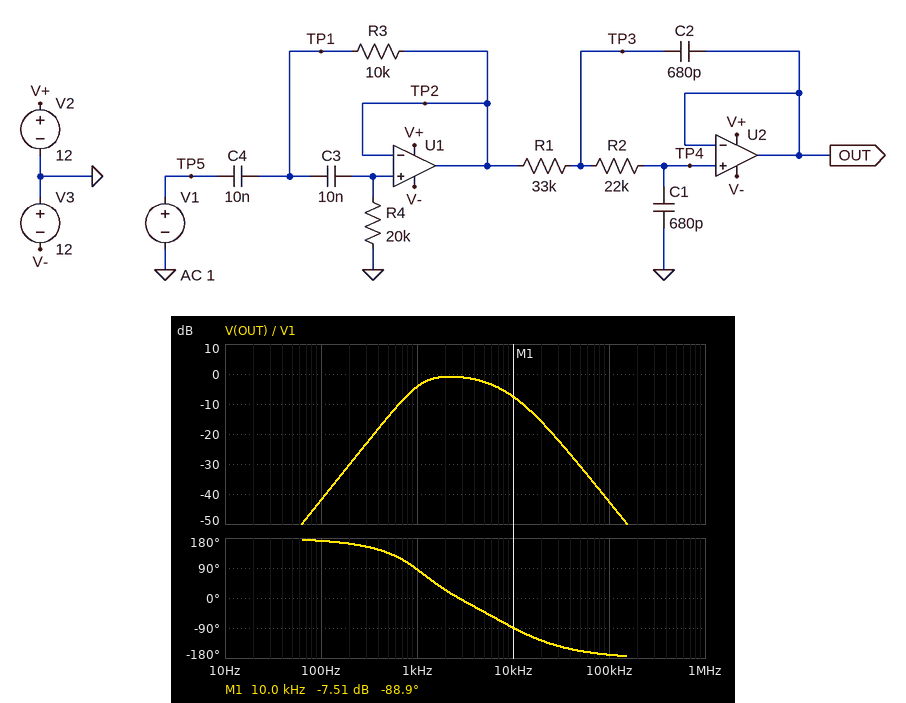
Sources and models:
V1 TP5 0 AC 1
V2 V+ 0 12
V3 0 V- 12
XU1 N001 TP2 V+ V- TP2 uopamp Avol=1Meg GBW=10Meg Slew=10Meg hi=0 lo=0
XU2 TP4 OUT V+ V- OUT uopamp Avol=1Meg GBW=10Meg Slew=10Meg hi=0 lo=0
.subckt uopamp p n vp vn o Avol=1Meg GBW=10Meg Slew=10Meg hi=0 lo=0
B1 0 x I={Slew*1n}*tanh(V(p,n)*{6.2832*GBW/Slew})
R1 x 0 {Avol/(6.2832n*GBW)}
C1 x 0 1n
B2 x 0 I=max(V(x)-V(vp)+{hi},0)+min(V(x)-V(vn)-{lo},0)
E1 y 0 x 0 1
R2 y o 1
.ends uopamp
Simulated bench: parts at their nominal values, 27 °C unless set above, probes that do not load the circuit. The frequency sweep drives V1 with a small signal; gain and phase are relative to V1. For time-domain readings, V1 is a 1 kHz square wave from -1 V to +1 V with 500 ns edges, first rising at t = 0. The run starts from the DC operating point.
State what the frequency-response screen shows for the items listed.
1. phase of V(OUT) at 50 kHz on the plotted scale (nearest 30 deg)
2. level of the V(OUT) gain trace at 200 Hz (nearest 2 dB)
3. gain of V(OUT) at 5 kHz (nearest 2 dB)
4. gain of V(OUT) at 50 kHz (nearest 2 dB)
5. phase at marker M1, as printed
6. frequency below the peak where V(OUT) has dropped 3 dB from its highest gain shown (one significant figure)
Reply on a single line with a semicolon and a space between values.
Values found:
-150 deg; -30 dB; -2 dB; -30 dB; -88.9 deg; 1 kHz
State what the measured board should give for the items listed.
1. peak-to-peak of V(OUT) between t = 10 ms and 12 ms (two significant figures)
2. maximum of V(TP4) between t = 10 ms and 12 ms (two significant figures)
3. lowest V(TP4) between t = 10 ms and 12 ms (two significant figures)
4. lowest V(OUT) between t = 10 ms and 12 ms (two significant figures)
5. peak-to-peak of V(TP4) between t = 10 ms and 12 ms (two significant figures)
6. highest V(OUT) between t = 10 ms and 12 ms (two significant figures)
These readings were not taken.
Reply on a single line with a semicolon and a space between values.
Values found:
2.8 V; 1.4 V; -1.4 V; -1.4 V; 2.8 V; 1.4 V
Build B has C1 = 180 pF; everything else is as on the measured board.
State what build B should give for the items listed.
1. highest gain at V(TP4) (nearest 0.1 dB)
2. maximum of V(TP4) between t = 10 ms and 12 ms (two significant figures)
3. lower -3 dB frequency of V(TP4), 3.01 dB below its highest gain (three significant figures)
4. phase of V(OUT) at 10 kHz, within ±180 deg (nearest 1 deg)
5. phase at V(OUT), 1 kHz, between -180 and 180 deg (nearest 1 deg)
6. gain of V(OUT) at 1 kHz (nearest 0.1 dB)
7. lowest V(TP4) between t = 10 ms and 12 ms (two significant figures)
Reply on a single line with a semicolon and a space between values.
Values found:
1.0 dB; 2.1 V; 1.28 kHz; -35 deg; 96 deg; -4.1 dB; -2.1 V
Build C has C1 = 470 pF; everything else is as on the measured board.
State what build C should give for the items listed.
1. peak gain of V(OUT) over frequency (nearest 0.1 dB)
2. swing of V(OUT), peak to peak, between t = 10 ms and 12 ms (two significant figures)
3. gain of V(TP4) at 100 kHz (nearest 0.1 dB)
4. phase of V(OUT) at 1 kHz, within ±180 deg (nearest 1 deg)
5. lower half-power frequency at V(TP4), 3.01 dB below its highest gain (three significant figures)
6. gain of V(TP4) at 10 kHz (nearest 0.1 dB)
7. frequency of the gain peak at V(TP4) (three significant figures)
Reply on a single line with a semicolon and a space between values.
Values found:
-0.4 dB; 3.2 V; -39.3 dB; 90 deg; 1.08 kHz; -4.2 dB; 2.66 kHz
